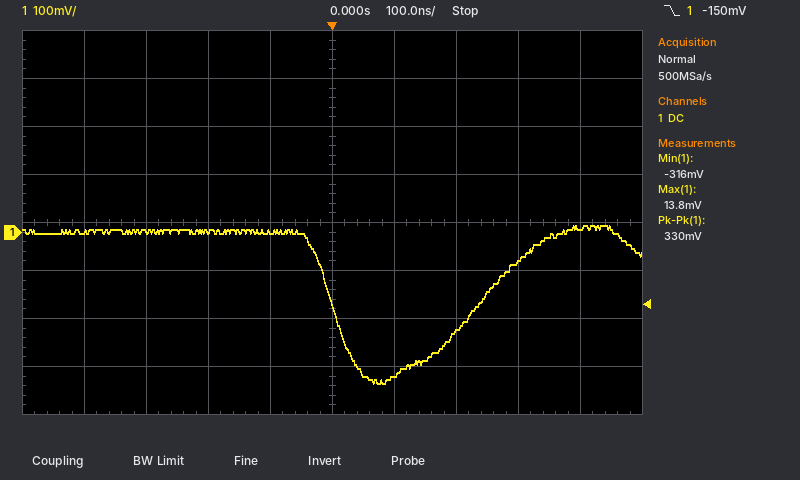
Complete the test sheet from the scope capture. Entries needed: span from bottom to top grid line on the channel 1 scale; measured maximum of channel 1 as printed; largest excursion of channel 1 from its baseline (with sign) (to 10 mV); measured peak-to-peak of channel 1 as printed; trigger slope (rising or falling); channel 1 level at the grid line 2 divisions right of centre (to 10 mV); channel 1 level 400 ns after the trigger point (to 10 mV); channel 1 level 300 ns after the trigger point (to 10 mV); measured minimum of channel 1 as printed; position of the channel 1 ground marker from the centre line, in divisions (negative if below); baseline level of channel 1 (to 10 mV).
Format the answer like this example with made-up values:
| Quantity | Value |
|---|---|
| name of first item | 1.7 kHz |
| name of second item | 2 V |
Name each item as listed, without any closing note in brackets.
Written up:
| Quantity | Value |
|---|---|
| span from bottom to top grid line on the channel 1 scale | 800 mV |
| measured maximum of channel 1 as printed | 13.8 mV |
| largest excursion of channel 1 from its baseline (with sign) | -320 mV |
| measured peak-to-peak of channel 1 as printed | 330 mV |
| trigger slope | falling |
| channel 1 level at the grid line 2 divisions right of centre | -210 mV |
| channel 1 level 400 ns after the trigger point | 10 mV |
| channel 1 level 300 ns after the trigger point | -60 mV |
| measured minimum of channel 1 as printed | -316 mV |
| position of the channel 1 ground marker from the centre line, in divisions | -0.2 div |
| baseline level of channel 1 | 0 mV |
